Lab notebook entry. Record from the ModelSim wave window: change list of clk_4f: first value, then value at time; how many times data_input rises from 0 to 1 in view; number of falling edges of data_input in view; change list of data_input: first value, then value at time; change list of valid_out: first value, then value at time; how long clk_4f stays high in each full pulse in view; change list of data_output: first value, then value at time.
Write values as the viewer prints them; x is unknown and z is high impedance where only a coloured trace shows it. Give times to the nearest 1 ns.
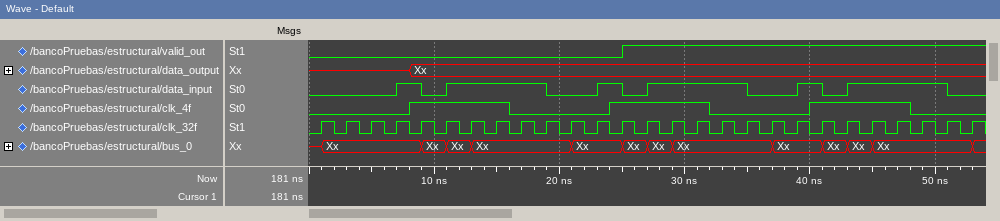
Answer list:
0, 1 at 8 ns, 0 at 16 ns, 1 at 24 ns, 0 at 32 ns, 1 at 40 ns, 0 at 48 ns
6
6
0, 1 at 7 ns, 0 at 9 ns, 1 at 11 ns, 0 at 19 ns, 1 at 23 ns, 0 at 25 ns, 1 at 27 ns, 0 at 35 ns, 1 at 39 ns, 0 at 41 ns, 1 at 43 ns, 0 at 51 ns
0, 1 at 25 ns
8 ns, 8 ns, 8 ns
x, Xx at 8 ns
